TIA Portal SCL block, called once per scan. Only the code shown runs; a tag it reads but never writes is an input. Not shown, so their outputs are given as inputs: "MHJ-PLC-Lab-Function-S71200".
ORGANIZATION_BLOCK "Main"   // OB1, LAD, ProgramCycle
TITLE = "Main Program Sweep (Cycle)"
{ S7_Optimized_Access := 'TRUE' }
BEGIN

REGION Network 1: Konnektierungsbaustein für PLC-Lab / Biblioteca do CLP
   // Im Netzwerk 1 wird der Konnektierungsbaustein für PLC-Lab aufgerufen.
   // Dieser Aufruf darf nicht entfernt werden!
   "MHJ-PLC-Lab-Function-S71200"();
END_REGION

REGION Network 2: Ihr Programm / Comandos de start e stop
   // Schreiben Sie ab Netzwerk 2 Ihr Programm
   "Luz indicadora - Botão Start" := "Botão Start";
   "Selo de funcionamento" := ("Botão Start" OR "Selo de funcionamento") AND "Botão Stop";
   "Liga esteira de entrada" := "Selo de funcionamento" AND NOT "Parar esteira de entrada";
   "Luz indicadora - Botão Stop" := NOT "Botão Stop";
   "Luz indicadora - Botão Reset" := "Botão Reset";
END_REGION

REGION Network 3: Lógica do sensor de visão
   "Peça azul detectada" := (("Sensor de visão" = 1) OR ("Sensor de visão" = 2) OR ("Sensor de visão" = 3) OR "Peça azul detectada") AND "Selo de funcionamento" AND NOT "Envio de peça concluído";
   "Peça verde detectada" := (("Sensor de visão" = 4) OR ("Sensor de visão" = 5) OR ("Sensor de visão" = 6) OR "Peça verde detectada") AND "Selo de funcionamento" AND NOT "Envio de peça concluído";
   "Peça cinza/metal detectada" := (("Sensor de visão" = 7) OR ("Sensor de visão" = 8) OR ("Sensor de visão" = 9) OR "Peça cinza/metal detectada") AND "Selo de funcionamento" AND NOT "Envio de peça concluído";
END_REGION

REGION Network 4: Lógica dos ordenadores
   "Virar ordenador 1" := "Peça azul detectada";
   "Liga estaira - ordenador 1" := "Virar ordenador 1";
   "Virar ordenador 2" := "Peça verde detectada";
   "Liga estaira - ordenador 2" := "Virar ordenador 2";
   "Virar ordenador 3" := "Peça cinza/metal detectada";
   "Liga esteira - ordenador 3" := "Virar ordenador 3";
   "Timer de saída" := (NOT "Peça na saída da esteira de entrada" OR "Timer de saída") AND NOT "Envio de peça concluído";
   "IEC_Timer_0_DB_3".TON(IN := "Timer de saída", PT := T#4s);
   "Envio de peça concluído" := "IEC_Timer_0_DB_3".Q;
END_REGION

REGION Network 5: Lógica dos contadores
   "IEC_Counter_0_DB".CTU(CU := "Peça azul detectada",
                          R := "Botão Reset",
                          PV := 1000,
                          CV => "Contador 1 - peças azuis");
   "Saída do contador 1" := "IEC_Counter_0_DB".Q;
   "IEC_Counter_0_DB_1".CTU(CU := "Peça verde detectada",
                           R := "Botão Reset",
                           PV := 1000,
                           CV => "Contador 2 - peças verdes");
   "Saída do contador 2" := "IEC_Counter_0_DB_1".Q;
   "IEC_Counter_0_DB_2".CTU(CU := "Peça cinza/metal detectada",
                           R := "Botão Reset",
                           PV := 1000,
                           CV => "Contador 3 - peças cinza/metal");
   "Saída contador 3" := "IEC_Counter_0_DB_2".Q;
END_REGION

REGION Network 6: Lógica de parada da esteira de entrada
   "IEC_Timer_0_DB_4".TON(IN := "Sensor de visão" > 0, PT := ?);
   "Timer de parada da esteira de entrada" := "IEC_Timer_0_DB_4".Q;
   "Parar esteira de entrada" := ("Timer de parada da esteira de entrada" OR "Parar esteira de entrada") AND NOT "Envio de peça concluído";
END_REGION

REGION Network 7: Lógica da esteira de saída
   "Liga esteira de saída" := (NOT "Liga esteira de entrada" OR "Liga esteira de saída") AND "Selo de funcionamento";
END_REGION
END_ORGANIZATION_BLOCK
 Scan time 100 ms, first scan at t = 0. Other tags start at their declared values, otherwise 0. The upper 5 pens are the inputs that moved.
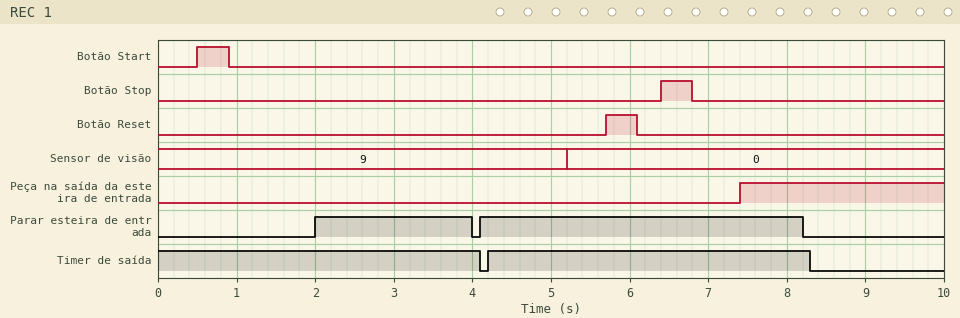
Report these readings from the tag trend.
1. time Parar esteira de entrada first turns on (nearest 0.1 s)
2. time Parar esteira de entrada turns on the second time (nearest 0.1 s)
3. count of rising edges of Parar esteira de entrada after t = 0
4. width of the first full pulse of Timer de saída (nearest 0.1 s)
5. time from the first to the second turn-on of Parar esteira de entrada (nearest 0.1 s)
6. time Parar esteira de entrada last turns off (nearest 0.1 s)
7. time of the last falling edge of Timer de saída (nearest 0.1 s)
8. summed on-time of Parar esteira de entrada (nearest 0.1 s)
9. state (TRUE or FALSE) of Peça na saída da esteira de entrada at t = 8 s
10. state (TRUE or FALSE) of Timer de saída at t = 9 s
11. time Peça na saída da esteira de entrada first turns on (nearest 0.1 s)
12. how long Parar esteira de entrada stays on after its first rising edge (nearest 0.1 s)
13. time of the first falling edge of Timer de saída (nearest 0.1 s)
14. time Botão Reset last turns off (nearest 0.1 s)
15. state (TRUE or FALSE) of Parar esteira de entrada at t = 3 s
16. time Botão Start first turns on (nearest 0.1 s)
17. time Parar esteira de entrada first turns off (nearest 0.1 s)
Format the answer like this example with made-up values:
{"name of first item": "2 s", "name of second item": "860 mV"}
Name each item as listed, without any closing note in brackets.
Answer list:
{"time Parar esteira de entrada first turns on": "2.0 s", "time Parar esteira de entrada turns on the second time": "4.1 s", "count of rising edges of Parar esteira de entrada after t = 0": "2", "width of the first full pulse of Timer de saída": "4.1 s", "time from the first to the second turn-on of Parar esteira de entrada": "2.1 s", "time Parar esteira de entrada last turns off": "8.2 s", "time of the last falling edge of Timer de saída": "8.3 s", "summed on-time of Parar esteira de entrada": "6.1 s", "state (TRUE or FALSE) of Peça na saída da esteira de entrada at t = 8 s": "TRUE", "state (TRUE or FALSE) of Timer de saída at t = 9 s": "FALSE", "time Peça na saída da esteira de entrada first turns on": "7.4 s", "how long Parar esteira de entrada stays on after its first rising edge": "2.0 s", "time of the first falling edge of Timer de saída": "4.1 s", "time Botão Reset last turns off": "6.1 s", "state (TRUE or FALSE) of Parar esteira de entrada at t = 3 s": "TRUE", "time Botão Start first turns on": "0.5 s", "time Parar esteira de entrada first turns off": "4.0 s"}
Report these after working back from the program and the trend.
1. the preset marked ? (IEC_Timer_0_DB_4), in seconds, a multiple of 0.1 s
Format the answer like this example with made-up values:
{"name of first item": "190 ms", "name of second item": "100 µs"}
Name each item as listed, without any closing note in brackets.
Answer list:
{"the preset marked ? (IEC_Timer_0_DB_4), in seconds, a multiple of 0.1 s": "2.0 s"}
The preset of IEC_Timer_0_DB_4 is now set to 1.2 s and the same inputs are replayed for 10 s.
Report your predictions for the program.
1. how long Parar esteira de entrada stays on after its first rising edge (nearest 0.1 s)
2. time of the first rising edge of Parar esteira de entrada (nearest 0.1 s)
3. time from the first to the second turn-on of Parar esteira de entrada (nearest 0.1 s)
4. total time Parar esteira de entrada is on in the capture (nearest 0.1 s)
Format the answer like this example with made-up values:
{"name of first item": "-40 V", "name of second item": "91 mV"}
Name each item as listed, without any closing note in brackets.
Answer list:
{"how long Parar esteira de entrada stays on after its first rising edge": "2.8 s", "time of the first rising edge of Parar esteira de entrada": "1.2 s", "time from the first to the second turn-on of Parar esteira de entrada": "2.9 s", "total time Parar esteira de entrada is on in the capture": "6.9 s"}
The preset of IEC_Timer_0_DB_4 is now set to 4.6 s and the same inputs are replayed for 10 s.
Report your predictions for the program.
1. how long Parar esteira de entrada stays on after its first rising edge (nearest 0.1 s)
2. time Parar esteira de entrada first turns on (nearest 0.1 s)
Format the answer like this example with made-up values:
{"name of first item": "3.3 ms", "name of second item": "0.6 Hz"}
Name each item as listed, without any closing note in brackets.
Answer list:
{"how long Parar esteira de entrada stays on after its first rising edge": "3.6 s", "time Parar esteira de entrada first turns on": "4.6 s"}
